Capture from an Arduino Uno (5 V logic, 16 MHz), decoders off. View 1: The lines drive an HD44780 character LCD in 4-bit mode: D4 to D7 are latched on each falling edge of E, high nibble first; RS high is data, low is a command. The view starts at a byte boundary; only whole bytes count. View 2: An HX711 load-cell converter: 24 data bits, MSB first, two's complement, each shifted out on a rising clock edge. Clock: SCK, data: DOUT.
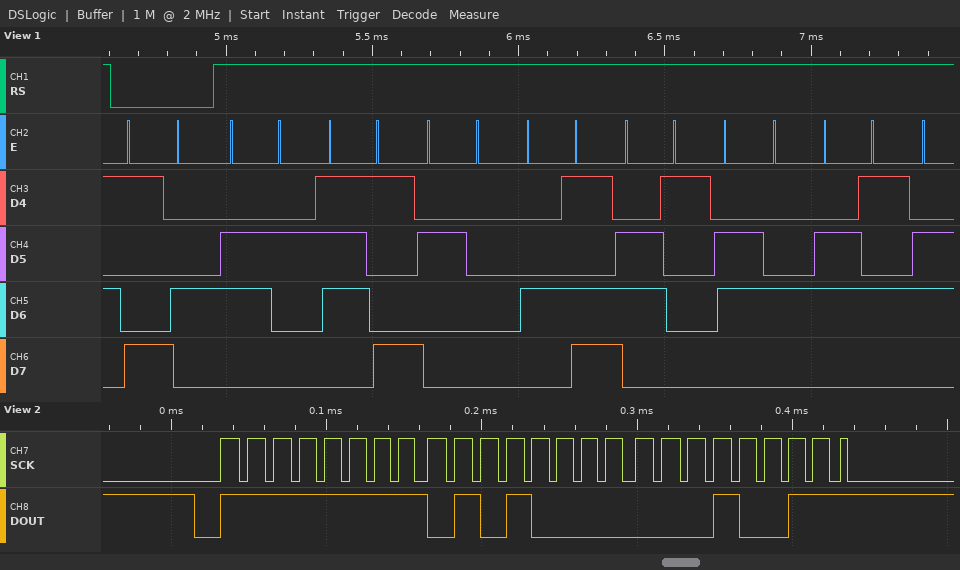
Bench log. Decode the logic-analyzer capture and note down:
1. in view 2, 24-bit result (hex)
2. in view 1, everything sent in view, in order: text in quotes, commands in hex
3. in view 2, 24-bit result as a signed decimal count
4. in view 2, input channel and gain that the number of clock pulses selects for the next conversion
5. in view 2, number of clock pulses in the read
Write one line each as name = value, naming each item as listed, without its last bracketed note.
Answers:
in view 2, 24-bit result = 0xFF5013
in view 1, everything sent in view, in order: text in quotes, commands in hex = 0x94 "by Made"
in view 2, 24-bit result as a signed decimal count = -45037
in view 2, input channel and gain that the number of clock pulses selects for the next conversion = channel A, gain 128
in view 2, number of clock pulses in the read = 25
